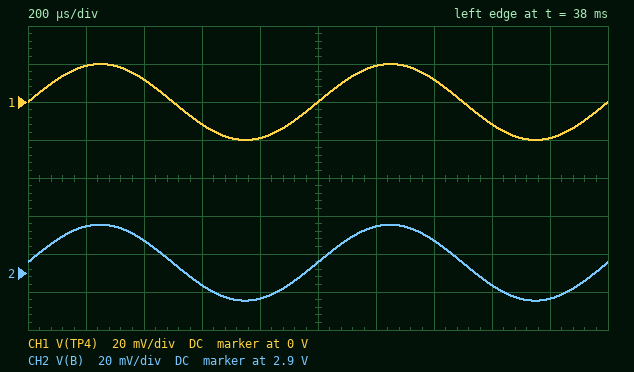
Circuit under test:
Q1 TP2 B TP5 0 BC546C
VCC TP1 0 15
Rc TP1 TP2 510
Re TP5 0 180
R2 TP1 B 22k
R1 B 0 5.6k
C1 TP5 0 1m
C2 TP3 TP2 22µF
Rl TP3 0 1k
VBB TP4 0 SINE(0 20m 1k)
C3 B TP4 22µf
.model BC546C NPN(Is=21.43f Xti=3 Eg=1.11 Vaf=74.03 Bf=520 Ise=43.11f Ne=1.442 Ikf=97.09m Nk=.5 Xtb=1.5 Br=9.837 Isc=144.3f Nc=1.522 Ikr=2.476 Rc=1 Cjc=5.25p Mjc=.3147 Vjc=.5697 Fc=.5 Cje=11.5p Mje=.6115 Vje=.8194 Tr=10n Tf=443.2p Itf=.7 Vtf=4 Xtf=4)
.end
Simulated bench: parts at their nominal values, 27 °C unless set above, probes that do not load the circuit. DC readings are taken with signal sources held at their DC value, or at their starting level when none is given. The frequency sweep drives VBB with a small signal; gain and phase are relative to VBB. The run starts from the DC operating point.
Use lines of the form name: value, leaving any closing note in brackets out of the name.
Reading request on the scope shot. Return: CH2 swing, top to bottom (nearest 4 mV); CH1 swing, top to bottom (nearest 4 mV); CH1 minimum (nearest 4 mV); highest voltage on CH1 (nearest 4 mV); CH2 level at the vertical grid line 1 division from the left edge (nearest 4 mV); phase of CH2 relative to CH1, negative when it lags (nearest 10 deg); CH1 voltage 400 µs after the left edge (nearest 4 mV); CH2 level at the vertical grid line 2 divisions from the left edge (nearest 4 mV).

CH2 swing, top to bottom: 40 mV
CH1 swing, top to bottom: 40 mV
CH1 minimum: -20 mV
highest voltage on CH1: 20 mV
CH2 level at the vertical grid line 1 division from the left edge: 2.924 V
phase of CH2 relative to CH1, negative when it lags: 0 deg
CH1 voltage 400 µs after the left edge: 12 mV
CH2 level at the vertical grid line 2 divisions from the left edge: 2.916 V
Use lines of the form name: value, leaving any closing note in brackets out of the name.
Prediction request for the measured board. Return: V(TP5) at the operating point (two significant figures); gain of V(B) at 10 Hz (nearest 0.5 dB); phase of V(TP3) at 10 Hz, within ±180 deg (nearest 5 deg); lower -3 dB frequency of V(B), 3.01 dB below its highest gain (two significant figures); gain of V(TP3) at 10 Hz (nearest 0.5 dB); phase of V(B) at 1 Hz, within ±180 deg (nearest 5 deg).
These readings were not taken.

V(TP5) at the operating point: 2.2 V
gain of V(B) at 10 Hz: -1.0 dB
phase of V(TP3) at 10 Hz, within ±180 deg: -70 deg
lower -3 dB frequency of V(B), 3.01 dB below its highest gain: 2.0 Hz
gain of V(TP3) at 10 Hz: 24.5 dB
phase of V(B) at 1 Hz, within ±180 deg: 55 deg
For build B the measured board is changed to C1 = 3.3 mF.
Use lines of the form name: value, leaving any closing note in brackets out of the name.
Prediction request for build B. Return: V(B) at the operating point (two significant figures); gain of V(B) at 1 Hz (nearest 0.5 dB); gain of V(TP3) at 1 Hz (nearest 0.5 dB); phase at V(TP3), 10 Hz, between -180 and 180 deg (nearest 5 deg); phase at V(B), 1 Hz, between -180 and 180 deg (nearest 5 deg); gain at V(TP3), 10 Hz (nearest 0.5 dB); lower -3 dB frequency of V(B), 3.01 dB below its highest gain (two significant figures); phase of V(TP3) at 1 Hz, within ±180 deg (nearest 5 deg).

V(B) at the operating point: 2.9 V
gain of V(B) at 1 Hz: -7.0 dB
gain of V(TP3) at 1 Hz: -4.0 dB
phase at V(TP3), 10 Hz, between -180 and 180 deg: -80 deg
phase at V(B), 1 Hz, between -180 and 180 deg: 50 deg
gain at V(TP3), 10 Hz: 32.0 dB
lower -3 dB frequency of V(B), 3.01 dB below its highest gain: 6.4 Hz
phase of V(TP3) at 1 Hz, within ±180 deg: 20 deg
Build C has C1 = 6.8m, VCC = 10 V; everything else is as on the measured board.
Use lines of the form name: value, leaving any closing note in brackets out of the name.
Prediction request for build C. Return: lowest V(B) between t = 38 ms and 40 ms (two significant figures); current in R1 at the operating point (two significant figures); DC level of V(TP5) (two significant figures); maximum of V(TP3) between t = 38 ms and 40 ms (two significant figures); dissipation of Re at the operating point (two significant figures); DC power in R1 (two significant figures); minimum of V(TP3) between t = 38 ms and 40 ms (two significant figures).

lowest V(B) between t = 38 ms and 40 ms: 1.9 V
current in R1 at the operating point: 350 µA
DC level of V(TP5): 1.3 V
maximum of V(TP3) between t = 38 ms and 40 ms: 1.4 V
dissipation of Re at the operating point: 8.9 mW
DC power in R1: 680 µW
minimum of V(TP3) between t = 38 ms and 40 ms: -1.8 V
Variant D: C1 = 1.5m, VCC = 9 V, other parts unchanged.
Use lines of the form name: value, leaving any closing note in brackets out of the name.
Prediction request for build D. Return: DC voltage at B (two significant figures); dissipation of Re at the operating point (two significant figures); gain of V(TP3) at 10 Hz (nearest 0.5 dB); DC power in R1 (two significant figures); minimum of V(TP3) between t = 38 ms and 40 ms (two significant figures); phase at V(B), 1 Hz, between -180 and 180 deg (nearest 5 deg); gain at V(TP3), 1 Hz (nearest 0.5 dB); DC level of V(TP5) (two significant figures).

DC voltage at B: 1.8 V
dissipation of Re at the operating point: 6.4 mW
gain of V(TP3) at 10 Hz: 27.0 dB
DC power in R1: 550 µW
minimum of V(TP3) between t = 38 ms and 40 ms: -1.6 V
phase at V(B), 1 Hz, between -180 and 180 deg: 55 deg
gain at V(TP3), 1 Hz: -9.0 dB
DC level of V(TP5): 1.1 V
